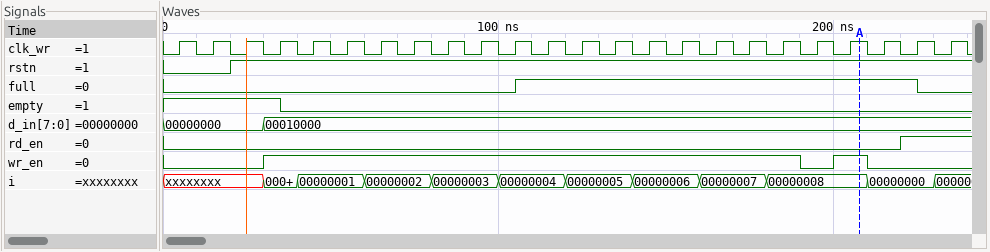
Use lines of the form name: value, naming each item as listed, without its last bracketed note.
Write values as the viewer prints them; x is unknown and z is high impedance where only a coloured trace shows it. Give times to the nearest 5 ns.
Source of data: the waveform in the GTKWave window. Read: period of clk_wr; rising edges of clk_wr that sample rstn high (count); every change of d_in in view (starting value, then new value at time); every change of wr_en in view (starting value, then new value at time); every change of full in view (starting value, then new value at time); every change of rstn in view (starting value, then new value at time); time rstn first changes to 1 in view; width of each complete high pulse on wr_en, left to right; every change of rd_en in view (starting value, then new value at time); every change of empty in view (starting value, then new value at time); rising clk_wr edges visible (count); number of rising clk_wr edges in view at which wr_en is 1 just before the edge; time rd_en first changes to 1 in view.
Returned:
period of clk_wr: 10 ns
rising edges of clk_wr that sample rstn high: 22
every change of d_in in view: 00000000, 00010000 at 30 ns
every change of wr_en in view: 0, 1 at 30 ns, 0 at 190 ns, 1 at 200 ns, 0 at 210 ns
every change of full in view: 0, 1 at 105 ns, 0 at 225 ns
every change of rstn in view: 0, 1 at 20 ns
time rstn first changes to 1 in view: 20 ns
width of each complete high pulse on wr_en, left to right: 160 ns, 10 ns
every change of rd_en in view: 0, 1 at 220 ns
every change of empty in view: 1, 0 at 35 ns
rising clk_wr edges visible: 24
number of rising clk_wr edges in view at which wr_en is 1 just before the edge: 17
time rd_en first changes to 1 in view: 220 ns
